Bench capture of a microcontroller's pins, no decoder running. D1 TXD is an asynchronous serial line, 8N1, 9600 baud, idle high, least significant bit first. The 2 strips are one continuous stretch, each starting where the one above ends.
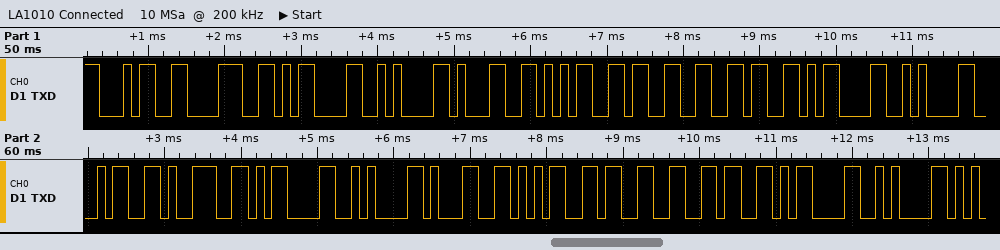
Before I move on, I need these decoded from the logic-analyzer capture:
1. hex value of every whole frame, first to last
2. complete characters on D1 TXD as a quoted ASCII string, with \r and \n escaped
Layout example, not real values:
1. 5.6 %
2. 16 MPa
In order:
1. 0x34 0x38 0x0D 0x0A 0x31 0x35 0x33 0x36 0x0D 0x0A 0x34 0x39 0x0D 0x0A 0x31 0x35 0x33 0x36 0x0D 0x0A
2. "48\r\n1536\r\n49\r\n1536\r\n"
